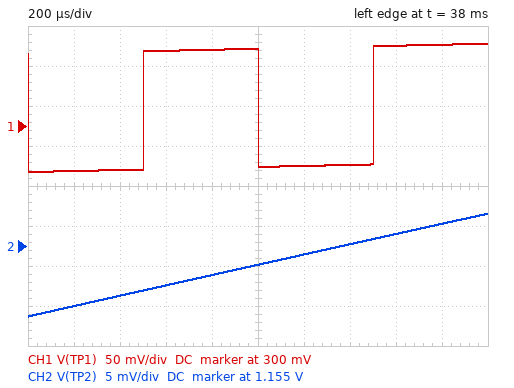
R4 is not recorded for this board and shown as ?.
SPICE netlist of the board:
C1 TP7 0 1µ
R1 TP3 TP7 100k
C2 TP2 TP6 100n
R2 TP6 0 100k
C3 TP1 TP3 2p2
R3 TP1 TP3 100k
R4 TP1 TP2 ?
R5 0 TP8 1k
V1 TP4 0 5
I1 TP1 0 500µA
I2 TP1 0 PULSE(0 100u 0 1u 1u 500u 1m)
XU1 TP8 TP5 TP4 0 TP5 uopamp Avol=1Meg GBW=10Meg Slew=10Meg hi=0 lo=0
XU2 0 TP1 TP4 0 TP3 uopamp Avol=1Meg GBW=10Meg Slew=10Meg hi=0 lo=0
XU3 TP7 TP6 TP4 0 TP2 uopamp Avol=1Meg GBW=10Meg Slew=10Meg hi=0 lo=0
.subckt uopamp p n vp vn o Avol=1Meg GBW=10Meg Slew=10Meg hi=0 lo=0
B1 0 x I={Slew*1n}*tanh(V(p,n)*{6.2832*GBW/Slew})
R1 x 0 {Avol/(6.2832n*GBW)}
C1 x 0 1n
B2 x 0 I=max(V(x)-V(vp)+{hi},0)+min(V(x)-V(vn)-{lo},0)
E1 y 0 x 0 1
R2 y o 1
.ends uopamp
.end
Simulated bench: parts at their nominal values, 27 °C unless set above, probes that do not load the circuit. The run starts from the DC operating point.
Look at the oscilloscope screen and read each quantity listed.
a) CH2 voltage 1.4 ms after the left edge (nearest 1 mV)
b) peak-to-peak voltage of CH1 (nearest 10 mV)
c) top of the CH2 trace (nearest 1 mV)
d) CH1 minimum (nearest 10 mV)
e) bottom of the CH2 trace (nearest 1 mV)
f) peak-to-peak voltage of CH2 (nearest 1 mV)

1.155 V
160 mV
1.159 V
240 mV
1.146 V
13 mV
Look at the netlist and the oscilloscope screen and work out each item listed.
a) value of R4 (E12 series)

1.5 kΩ
